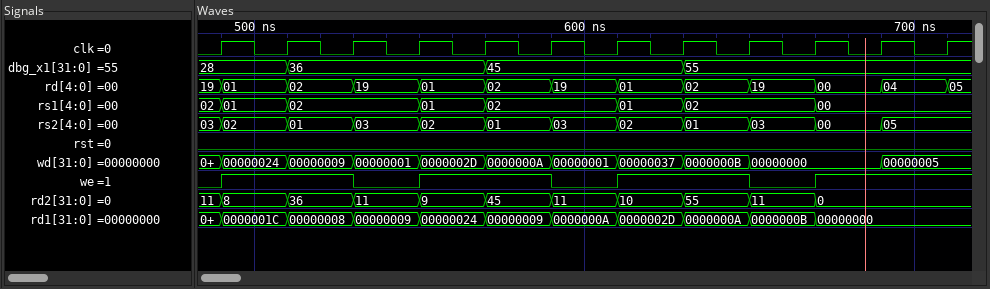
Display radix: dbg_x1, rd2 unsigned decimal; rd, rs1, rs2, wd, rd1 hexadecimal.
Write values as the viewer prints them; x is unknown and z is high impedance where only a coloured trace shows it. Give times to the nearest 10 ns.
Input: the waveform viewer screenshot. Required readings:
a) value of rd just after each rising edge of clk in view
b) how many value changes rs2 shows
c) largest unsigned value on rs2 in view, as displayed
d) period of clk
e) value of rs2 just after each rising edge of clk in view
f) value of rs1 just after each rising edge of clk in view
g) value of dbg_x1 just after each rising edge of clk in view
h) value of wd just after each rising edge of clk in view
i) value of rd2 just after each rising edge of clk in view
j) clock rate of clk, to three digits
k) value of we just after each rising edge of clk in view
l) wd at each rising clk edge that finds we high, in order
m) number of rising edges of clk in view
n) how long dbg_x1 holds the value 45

01, 02, 19, 01, 02, 19, 01, 02, 19, 00, 04, 05
11
05
20 ns
02, 01, 03, 02, 01, 03, 02, 01, 03, 00, 05, 05
01, 02, 02, 01, 02, 02, 01, 02, 02, 00, 00, 00
28, 36, 36, 36, 45, 45, 45, 55, 55, 55, 55, 55
00000024, 00000009, 00000001, 0000002D, 0000000A, 00000001, 00000037, 0000000B, 00000000, 00000000, 00000005, 00000005
8, 36, 11, 9, 45, 11, 10, 55, 11, 0, 0, 0
50.0 MHz
1 1 0 1 1 0 1 1 0 1 1 1
00000024, 00000009, 0000002D, 0000000A, 00000037, 0000000B, 00000000, 00000005
12
60 ns
